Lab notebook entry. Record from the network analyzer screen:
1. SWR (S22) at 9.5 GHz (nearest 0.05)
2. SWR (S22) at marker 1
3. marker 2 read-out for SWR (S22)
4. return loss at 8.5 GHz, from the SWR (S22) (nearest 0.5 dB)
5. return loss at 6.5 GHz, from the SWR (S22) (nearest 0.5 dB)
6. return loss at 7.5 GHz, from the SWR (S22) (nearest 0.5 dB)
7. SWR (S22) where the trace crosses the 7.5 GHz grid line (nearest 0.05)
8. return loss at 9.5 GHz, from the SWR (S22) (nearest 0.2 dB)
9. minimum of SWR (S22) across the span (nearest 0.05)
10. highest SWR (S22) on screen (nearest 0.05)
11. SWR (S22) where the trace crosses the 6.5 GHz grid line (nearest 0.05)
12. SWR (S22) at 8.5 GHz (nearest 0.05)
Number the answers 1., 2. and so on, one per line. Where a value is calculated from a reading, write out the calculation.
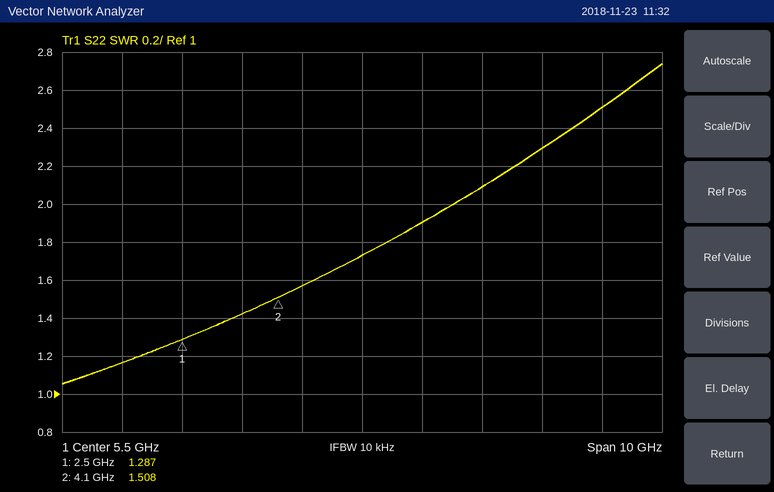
1. 2.50
2. 1.287
3. 1.508
4. −20 log10((2.3 − 1)/(2.3 + 1)) ≈ 8.09 dB, so 8.0 dB to the nearest 0.5 dB
5. −20 log10((1.9 − 1)/(1.9 + 1)) ≈ 10.2 dB, so 10.0 dB to the nearest 0.5 dB
6. −20 log10((2.1 − 1)/(2.1 + 1)) ≈ 9.0 dB
7. 2.10
8. −20 log10((2.5 − 1)/(2.5 + 1)) ≈ 7.4 dB
9. 1.05
10. 2.75
11. 1.90
12. 2.30
